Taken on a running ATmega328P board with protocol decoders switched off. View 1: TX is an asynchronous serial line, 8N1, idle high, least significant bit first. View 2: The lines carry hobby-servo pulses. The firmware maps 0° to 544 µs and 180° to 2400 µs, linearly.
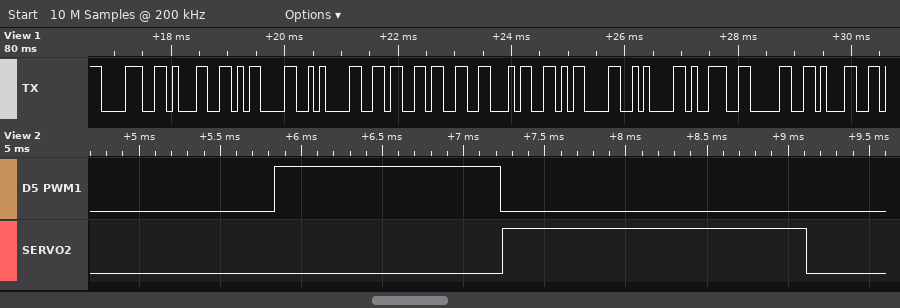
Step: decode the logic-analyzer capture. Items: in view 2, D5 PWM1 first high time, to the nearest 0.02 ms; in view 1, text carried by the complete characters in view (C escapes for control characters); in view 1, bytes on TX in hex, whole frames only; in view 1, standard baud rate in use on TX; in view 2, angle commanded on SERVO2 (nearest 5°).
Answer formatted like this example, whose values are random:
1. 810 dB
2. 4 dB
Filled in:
1. 1.40 ms
2. "81\r\n634\r\n901"
3. 38 31 0D 0A 36 33 34 0D 0A 39 30 31
4. 9600 baud
5. 130°
